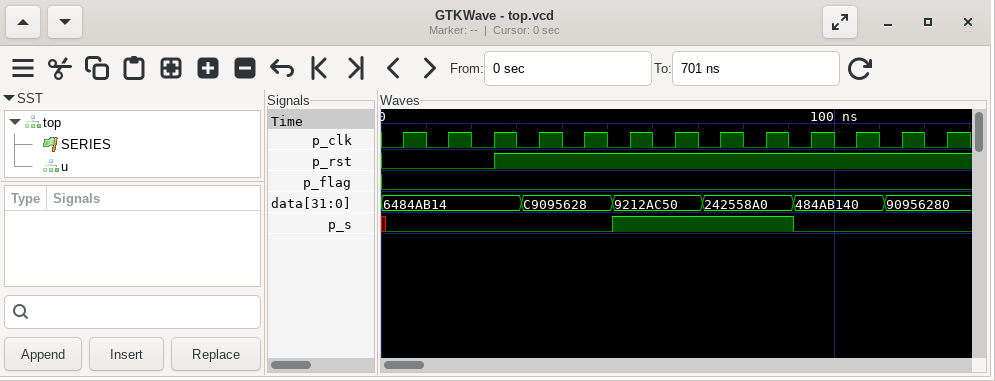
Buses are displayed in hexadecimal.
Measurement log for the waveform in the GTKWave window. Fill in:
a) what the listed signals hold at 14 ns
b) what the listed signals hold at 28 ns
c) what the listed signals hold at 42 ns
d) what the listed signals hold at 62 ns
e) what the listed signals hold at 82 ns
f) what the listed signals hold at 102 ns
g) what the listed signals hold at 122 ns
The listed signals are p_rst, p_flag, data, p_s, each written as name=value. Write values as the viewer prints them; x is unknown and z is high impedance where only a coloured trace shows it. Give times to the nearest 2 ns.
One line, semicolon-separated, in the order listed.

p_rst=0, p_flag=0, data=6484AB14, p_s=0; p_rst=1, p_flag=0, data=6484AB14, p_s=0; p_rst=1, p_flag=0, data=C9095628, p_s=0; p_rst=1, p_flag=0, data=9212AC50, p_s=1; p_rst=1, p_flag=0, data=242558A0, p_s=1; p_rst=1, p_flag=0, data=484AB140, p_s=0; p_rst=1, p_flag=0, data=90956280, p_s=0
